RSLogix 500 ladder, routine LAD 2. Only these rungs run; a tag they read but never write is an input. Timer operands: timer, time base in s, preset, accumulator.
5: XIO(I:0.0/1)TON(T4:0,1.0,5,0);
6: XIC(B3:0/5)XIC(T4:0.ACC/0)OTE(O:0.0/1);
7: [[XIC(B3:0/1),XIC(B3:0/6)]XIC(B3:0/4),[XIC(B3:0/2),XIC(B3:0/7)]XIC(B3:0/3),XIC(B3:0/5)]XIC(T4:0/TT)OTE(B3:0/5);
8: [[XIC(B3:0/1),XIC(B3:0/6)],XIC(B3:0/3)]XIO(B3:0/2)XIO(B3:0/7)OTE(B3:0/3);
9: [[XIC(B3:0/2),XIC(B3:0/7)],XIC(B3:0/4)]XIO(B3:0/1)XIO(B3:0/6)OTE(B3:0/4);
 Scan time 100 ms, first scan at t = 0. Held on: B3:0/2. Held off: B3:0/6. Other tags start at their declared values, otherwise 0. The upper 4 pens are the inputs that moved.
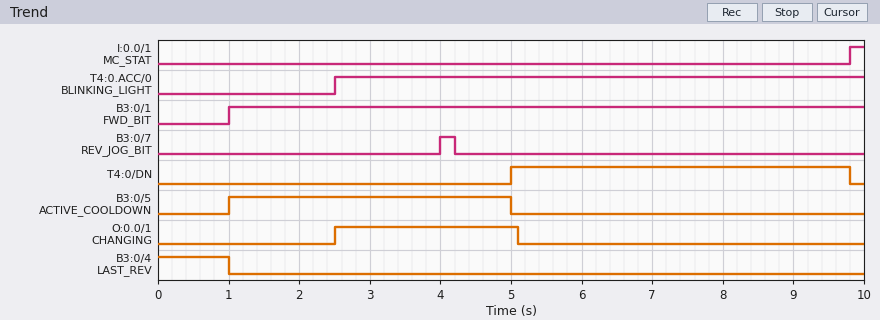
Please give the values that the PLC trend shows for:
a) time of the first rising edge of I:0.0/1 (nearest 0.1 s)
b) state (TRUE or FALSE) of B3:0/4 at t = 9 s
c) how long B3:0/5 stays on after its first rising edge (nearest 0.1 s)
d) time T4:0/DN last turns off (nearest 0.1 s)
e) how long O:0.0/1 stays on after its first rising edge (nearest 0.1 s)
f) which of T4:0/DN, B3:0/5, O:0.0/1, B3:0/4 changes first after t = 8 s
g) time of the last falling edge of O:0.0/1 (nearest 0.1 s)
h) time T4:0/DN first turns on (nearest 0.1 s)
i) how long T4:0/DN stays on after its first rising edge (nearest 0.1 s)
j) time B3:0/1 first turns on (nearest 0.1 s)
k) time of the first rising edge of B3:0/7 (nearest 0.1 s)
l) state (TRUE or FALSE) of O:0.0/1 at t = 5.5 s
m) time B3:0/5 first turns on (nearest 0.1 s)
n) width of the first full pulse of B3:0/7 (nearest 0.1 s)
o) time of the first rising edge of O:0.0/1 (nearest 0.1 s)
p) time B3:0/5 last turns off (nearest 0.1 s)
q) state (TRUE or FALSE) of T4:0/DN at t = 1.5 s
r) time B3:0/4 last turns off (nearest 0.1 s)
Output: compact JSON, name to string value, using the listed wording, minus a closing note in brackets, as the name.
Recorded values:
{"time of the first rising edge of I:0.0/1": "9.8 s", "state (TRUE or FALSE) of B3:0/4 at t = 9 s": "FALSE", "how long B3:0/5 stays on after its first rising edge": "4.0 s", "time T4:0/DN last turns off": "9.8 s", "how long O:0.0/1 stays on after its first rising edge": "2.6 s", "which of T4:0/DN, B3:0/5, O:0.0/1, B3:0/4 changes first after t = 8 s": "T4:0/DN", "time of the last falling edge of O:0.0/1": "5.1 s", "time T4:0/DN first turns on": "5.0 s", "how long T4:0/DN stays on after its first rising edge": "4.8 s", "time B3:0/1 first turns on": "1.0 s", "time of the first rising edge of B3:0/7": "4.0 s", "state (TRUE or FALSE) of O:0.0/1 at t = 5.5 s": "FALSE", "time B3:0/5 first turns on": "1.0 s", "width of the first full pulse of B3:0/7": "0.2 s", "time of the first rising edge of O:0.0/1": "2.5 s", "time B3:0/5 last turns off": "5.0 s", "state (TRUE or FALSE) of T4:0/DN at t = 1.5 s": "FALSE", "time B3:0/4 last turns off": "1.0 s"}
